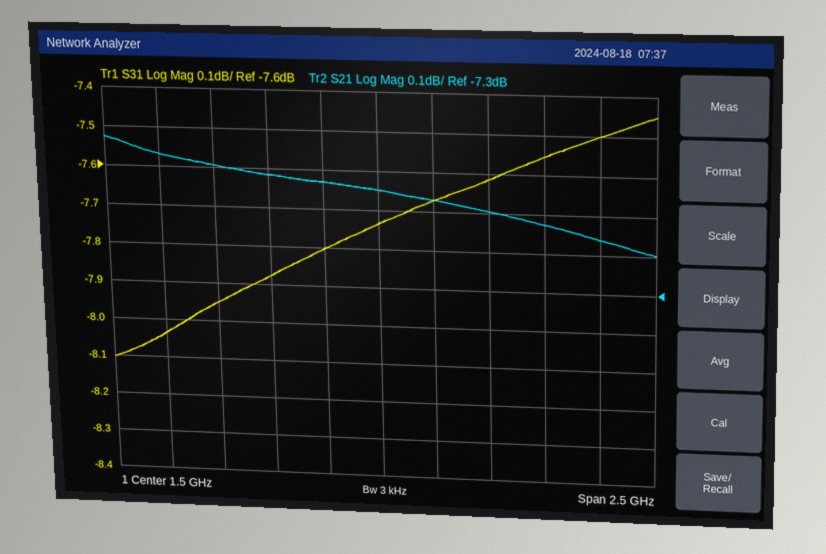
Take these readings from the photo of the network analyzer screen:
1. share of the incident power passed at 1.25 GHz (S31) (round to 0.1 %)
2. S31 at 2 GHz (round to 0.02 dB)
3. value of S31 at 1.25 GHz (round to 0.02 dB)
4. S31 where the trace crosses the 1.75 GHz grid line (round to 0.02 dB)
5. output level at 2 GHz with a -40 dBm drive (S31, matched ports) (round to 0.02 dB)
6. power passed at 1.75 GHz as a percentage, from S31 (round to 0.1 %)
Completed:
16.6 %
-7.62 dB
-7.80 dB
-7.68 dB
-47.62 dBm
17.1 %
